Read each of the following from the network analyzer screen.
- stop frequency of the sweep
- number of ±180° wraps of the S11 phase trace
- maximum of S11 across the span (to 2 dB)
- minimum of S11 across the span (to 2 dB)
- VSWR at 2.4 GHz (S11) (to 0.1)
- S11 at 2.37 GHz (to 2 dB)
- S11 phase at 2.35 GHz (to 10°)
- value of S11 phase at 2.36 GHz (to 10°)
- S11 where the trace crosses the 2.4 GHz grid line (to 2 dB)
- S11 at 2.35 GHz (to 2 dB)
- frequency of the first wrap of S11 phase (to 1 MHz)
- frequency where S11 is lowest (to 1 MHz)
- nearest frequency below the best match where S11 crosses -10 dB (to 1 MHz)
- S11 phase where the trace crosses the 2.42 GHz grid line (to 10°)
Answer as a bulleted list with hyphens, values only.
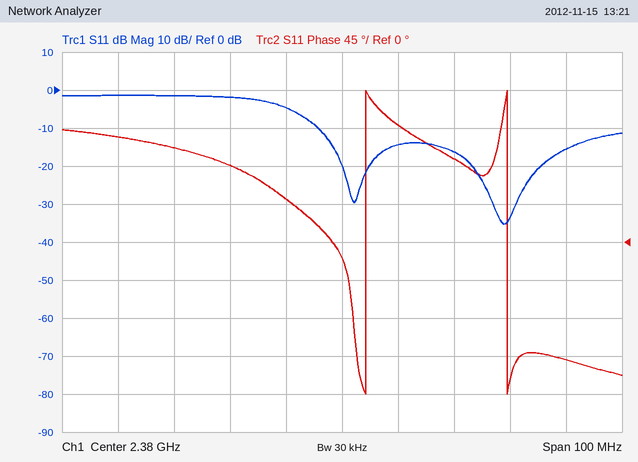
- 2.43 GHz
- 2
- -2 dB
- -36 dB
- 1.4
- -4 dB
- 110°
- 90°
- -16 dB
- -2 dB
- 2.384 GHz
- 2.409 GHz
- 2.376 GHz
- -140°
